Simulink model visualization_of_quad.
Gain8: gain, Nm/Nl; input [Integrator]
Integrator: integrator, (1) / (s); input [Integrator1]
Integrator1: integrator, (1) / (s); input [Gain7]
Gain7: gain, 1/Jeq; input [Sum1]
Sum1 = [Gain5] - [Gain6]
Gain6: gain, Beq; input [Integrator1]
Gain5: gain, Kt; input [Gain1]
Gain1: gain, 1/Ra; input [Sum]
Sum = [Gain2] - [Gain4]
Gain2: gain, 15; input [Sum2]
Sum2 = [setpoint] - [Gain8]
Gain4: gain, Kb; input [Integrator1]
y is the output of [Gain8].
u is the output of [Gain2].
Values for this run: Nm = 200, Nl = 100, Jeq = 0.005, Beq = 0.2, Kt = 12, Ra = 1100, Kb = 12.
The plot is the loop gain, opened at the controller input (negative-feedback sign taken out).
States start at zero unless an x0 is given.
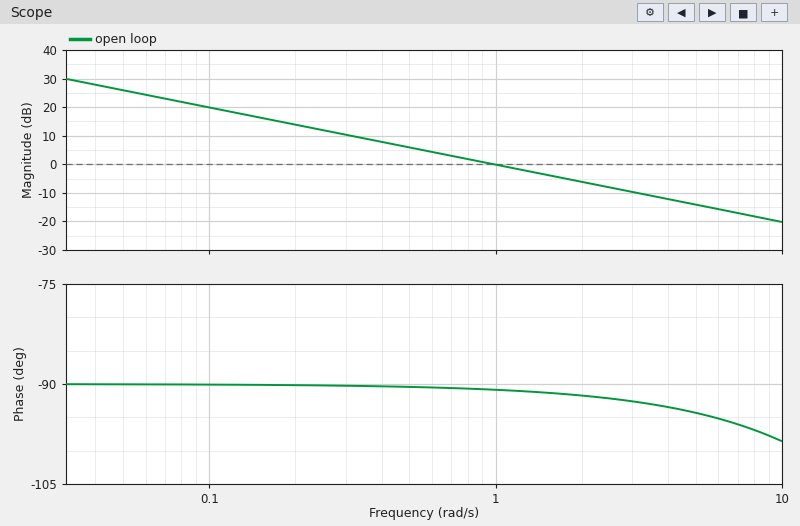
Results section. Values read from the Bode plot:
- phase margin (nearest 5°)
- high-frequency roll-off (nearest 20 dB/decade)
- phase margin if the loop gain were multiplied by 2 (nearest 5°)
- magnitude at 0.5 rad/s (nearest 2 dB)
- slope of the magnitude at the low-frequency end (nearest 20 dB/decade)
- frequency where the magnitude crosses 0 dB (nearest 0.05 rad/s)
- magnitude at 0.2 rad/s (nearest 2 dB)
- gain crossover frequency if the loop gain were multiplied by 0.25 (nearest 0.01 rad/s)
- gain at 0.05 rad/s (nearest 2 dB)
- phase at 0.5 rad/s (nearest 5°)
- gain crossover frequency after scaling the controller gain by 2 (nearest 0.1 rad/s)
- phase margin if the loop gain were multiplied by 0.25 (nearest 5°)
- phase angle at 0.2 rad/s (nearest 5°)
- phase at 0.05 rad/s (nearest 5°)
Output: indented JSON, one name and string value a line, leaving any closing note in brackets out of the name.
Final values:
{
  "phase margin": "90°",
  "high-frequency roll-off": "-20 dB/decade",
  "phase margin if the loop gain were multiplied by 2": "90°",
  "magnitude at 0.5 rad/s": "6 dB",
  "slope of the magnitude at the low-frequency end": "-20 dB/decade",
  "frequency where the magnitude crosses 0 dB": "1.00 rad/s",
  "magnitude at 0.2 rad/s": "14 dB",
  "gain crossover frequency if the loop gain were multiplied by 0.25": "0.25 rad/s",
  "gain at 0.05 rad/s": "26 dB",
  "phase at 0.5 rad/s": "-90°",
  "gain crossover frequency after scaling the controller gain by 2": "2.0 rad/s",
  "phase margin if the loop gain were multiplied by 0.25": "90°",
  "phase angle at 0.2 rad/s": "-90°",
  "phase at 0.05 rad/s": "-90°"
}
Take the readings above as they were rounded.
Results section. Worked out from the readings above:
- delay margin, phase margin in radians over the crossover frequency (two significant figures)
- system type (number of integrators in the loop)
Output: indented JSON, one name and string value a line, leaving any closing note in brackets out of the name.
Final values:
{
  "delay margin, phase margin in radians over the crossover frequency": "1.6 s",
  "system type": "1"
}
